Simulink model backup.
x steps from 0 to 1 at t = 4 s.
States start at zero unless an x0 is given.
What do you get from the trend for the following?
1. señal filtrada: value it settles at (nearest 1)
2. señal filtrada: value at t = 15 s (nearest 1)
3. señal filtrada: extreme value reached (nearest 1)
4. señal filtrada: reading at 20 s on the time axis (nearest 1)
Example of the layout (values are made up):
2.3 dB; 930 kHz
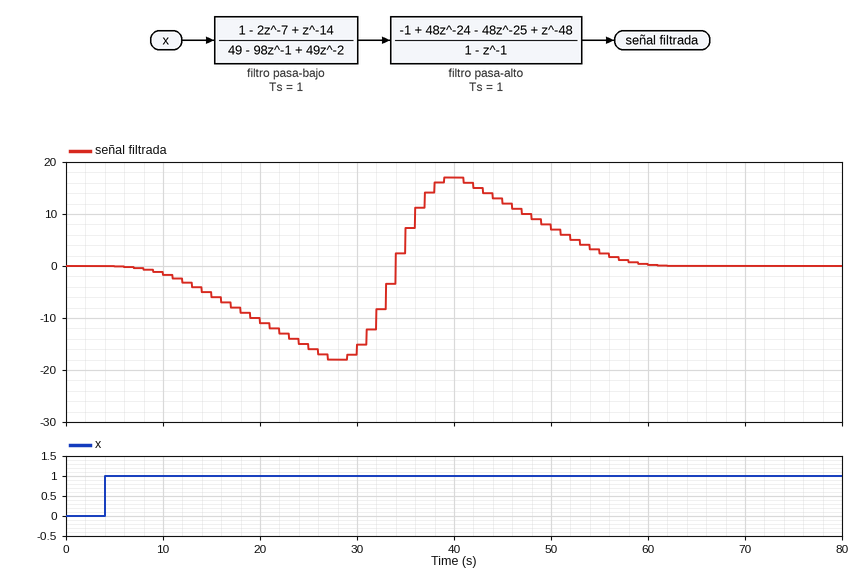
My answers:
0; -6; -18; -11
